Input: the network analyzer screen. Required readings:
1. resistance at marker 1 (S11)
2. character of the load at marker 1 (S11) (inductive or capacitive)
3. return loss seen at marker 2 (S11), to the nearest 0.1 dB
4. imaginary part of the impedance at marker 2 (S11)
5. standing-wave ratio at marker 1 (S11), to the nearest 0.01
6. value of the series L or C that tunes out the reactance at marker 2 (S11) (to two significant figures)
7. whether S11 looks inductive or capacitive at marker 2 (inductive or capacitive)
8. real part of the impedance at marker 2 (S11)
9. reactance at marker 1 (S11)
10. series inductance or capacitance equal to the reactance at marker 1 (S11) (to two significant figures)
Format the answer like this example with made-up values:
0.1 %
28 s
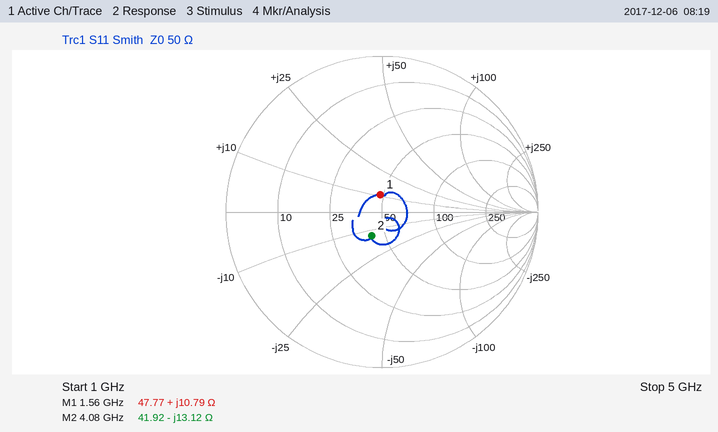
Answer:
47.77 Ω
inductive
15.6 dB
-13.12 Ω
1.25
510 pH
capacitive
41.92 Ω
+10.79 Ω
1.1 nH
